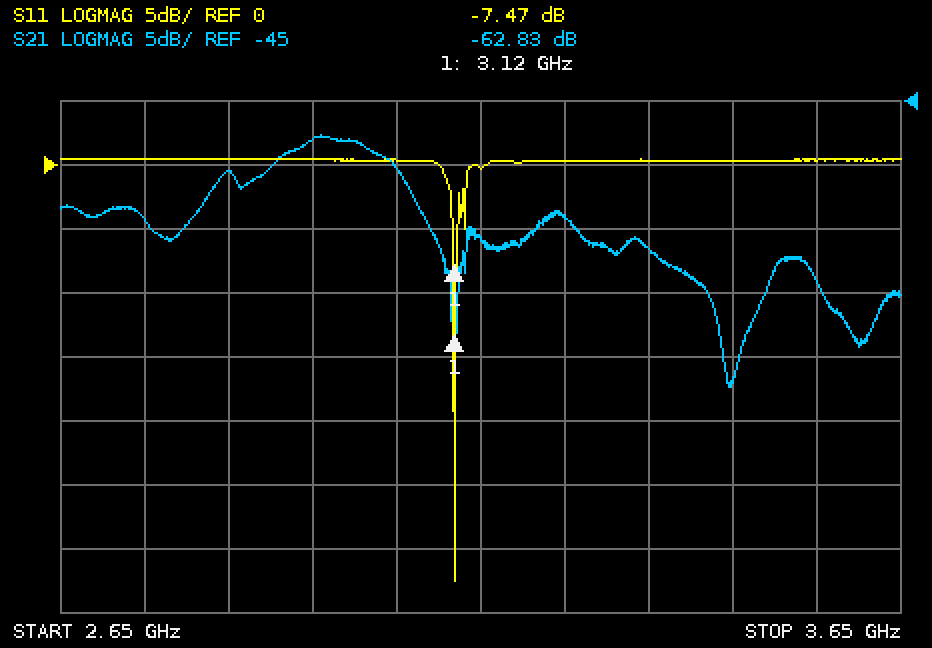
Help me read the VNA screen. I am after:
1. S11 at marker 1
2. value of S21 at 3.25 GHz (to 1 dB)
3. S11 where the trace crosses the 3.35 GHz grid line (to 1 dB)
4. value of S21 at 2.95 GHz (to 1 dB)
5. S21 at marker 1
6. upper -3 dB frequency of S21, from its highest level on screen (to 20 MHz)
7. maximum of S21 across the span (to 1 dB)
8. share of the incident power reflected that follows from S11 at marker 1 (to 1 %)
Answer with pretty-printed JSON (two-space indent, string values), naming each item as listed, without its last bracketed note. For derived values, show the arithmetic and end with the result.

{
  "S11 at marker 1": "-7.47 dB",
  "value of S21 at 3.25 GHz": "-54 dB",
  "S11 where the trace crosses the 3.35 GHz grid line": "0 dB",
  "value of S21 at 2.95 GHz": "-48 dB",
  "S21 at marker 1": "-62.83 dB",
  "upper -3 dB frequency of S21, from its highest level on screen": "3.06 GHz",
  "maximum of S21 across the span": "-48 dB",
  "share of the incident power reflected that follows from S11 at marker 1": "10^(-7.47/10) ≈ 18 %"
}
